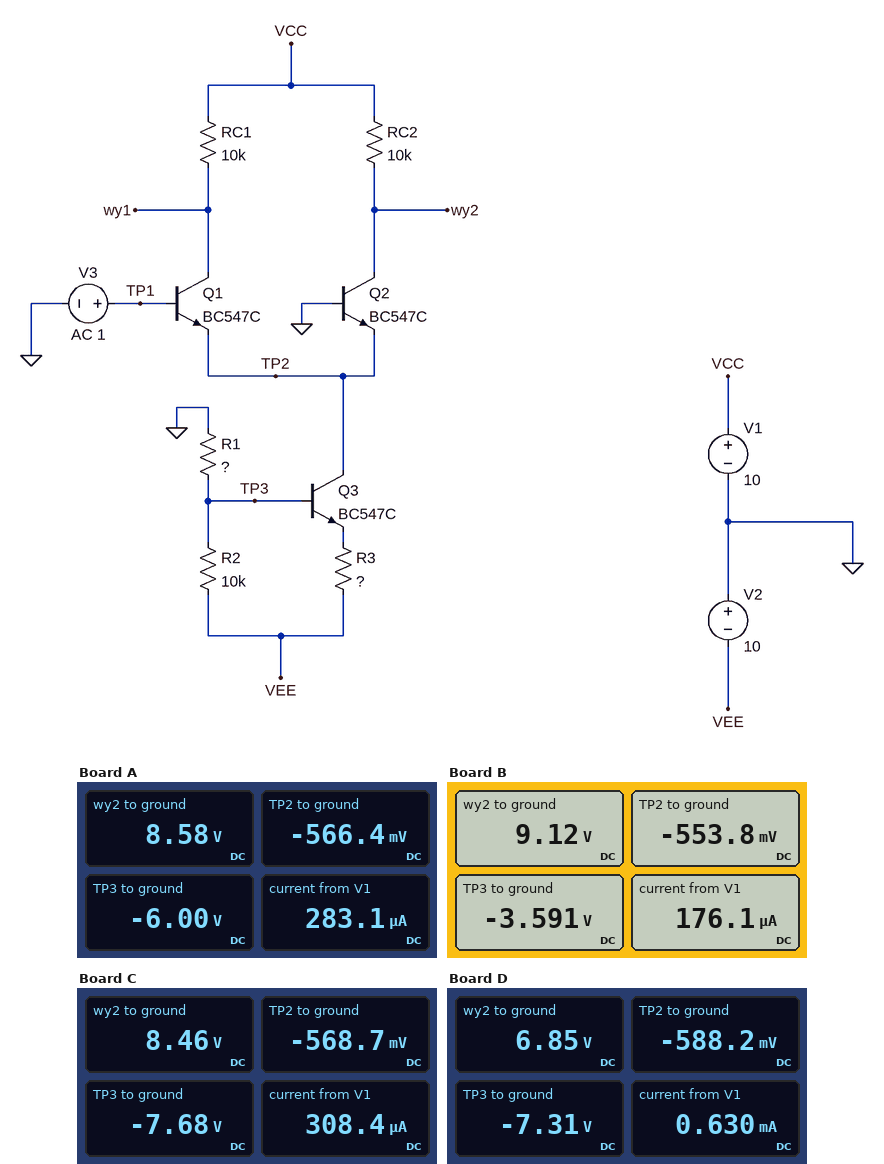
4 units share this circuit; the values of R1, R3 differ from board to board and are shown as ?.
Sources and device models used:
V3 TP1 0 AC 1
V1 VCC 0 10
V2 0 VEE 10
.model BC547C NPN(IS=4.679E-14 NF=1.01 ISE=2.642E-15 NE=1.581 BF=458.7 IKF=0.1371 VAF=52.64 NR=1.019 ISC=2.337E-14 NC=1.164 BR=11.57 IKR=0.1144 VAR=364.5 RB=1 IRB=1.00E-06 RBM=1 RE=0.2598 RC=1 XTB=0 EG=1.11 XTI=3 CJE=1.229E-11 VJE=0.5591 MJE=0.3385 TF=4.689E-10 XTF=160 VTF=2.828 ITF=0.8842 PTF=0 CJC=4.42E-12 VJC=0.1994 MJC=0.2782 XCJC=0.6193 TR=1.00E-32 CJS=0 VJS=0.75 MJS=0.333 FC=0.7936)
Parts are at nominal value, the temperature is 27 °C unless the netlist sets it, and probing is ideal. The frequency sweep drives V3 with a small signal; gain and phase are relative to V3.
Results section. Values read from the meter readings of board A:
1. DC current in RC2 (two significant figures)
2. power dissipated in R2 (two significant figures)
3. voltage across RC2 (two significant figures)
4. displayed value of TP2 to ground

140 µA
1.6 mW
1.4 V
-566.4 mV
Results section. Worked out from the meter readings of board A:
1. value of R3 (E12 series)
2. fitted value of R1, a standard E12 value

12 kΩ
15 kΩ
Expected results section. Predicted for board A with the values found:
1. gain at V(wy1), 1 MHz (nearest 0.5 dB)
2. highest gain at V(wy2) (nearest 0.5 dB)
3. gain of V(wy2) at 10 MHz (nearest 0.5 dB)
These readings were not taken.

28.5 dB
28.5 dB
25.5 dB
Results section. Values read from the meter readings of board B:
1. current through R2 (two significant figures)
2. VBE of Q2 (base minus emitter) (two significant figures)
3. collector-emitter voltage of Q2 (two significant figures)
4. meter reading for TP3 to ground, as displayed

640 µA
550 mV
9.7 V
-3.591 V
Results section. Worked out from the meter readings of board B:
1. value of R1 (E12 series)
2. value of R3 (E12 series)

5.6 kΩ
33 kΩ
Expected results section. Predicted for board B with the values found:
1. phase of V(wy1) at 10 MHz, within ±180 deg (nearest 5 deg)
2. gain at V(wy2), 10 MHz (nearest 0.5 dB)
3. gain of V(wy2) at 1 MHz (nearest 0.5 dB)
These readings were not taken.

135 deg
21.5 dB
24.5 dB
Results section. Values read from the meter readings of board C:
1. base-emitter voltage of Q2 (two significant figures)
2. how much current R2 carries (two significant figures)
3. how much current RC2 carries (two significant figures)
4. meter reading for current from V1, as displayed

570 mV
230 µA
150 µA
308.4 µA
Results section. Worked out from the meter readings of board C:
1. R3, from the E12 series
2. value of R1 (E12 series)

5.6 kΩ
33 kΩ
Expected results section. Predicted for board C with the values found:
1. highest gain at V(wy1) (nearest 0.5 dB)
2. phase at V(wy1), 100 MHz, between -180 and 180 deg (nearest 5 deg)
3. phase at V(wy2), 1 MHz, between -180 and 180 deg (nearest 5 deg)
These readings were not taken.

29.0 dB
75 deg
-5 deg
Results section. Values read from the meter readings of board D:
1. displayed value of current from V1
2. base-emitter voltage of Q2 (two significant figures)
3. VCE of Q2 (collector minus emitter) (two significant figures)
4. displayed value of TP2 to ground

0.630 mA
590 mV
7.4 V
-588.2 mV
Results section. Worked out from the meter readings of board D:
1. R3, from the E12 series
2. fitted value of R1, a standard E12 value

3.3 kΩ
27 kΩ
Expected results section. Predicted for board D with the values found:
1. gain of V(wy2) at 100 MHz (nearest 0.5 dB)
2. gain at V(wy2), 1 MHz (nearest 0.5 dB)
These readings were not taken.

15.0 dB
35.0 dB
